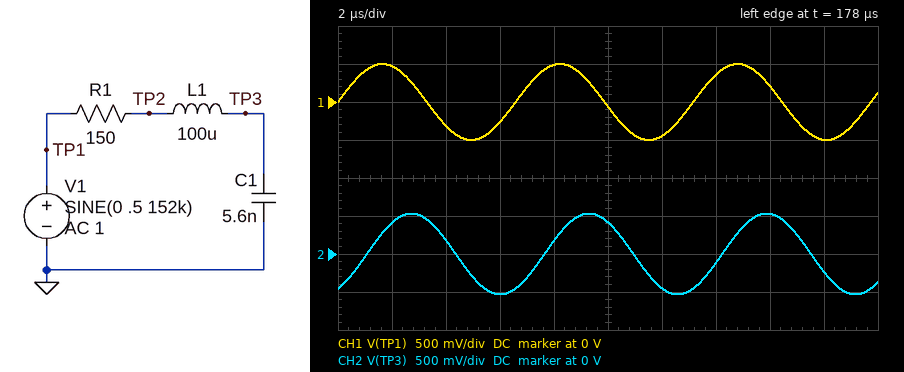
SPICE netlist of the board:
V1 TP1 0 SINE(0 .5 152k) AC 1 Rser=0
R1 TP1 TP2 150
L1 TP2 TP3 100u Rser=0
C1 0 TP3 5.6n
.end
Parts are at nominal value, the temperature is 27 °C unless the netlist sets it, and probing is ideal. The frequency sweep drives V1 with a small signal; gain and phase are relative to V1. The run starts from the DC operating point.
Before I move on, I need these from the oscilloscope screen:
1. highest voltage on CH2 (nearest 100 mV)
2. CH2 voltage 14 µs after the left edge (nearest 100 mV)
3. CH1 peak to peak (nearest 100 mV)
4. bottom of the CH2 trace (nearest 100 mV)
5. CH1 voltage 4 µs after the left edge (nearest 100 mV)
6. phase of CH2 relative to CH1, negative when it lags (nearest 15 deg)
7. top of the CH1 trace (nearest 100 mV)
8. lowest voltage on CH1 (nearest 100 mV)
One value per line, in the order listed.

500 mV
-100 mV
1.0 V
-500 mV
-300 mV
-60 deg
500 mV
-500 mV
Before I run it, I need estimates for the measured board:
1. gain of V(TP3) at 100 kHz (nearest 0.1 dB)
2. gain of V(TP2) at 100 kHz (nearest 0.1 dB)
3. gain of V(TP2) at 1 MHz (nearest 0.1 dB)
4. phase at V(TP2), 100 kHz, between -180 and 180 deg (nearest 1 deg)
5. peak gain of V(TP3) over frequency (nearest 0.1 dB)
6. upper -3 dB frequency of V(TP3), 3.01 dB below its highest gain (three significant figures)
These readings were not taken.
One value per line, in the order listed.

0.5 dB
-1.6 dB
-0.3 dB
-34 deg
0.6 dB
242 kHz
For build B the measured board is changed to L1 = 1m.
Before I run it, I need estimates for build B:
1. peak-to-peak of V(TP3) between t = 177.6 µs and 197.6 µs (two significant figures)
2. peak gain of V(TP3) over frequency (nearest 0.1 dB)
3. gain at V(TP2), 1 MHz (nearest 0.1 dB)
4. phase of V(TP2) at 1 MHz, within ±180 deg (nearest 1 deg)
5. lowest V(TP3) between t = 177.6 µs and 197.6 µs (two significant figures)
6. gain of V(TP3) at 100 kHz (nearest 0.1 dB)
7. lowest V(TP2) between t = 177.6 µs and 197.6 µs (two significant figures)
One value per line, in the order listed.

240 mV
9.1 dB
0 dB
1 deg
-120 mV
-2.4 dB
-490 mV
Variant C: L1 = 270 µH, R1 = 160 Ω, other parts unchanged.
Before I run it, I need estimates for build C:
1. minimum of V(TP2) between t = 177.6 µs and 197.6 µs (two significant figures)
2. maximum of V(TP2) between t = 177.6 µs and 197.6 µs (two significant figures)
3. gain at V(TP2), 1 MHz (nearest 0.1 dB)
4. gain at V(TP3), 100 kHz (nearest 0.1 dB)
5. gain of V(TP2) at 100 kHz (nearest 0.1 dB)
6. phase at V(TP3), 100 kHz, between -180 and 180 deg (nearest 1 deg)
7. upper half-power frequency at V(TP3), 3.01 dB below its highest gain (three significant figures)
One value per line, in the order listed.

-200 mV
200 mV
0 dB
3.2 dB
-4.7 dB
-54 deg
154 kHz
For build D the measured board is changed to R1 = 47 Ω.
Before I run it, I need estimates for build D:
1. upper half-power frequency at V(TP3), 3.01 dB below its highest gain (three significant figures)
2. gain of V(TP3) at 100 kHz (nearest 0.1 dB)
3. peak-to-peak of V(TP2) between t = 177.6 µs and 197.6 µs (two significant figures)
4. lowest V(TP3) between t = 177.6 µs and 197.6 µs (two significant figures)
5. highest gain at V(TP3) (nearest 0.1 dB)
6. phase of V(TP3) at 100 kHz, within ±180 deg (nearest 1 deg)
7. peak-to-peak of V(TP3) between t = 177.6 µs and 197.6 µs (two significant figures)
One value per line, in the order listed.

241 kHz
2.0 dB
890 mV
-910 mV
9.2 dB
-12 deg
1.8 V
